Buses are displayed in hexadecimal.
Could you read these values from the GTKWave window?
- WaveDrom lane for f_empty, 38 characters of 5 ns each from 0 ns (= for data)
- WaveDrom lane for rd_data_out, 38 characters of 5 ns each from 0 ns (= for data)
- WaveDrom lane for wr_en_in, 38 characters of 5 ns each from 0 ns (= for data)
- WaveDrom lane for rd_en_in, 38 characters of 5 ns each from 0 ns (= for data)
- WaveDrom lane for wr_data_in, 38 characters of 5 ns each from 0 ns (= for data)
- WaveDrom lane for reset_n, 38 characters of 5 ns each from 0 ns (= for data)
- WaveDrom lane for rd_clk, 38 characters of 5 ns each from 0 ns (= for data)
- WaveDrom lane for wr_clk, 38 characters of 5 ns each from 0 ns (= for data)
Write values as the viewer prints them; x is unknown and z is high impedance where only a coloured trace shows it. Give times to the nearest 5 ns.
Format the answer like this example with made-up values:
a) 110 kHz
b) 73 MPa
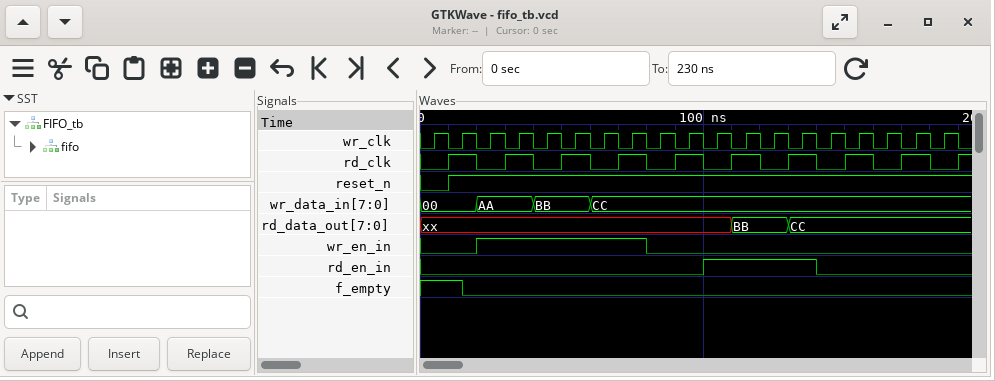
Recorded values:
a) {name: 'f_empty', wave: '1..0..................................'}
b) {name: 'rd_data_out', wave: 'x.....................=...=...........', data: 'BB CC'}
c) {name: 'wr_en_in', wave: '0...1...........0.....................'}
d) {name: 'rd_en_in', wave: '0...................1.......0.........'}
e) {name: 'wr_data_in', wave: '=...=...=...=.........................', data: '00 AA BB CC'}
f) {name: 'reset_n', wave: '0.1...................................'}
g) {name: 'rd_clk', wave: '0.1.0.1.0.1.0.1.0.1.0.1.0.1.0.1.0.1.0.'}
h) {name: 'wr_clk', wave: '01010101010101010101010101010101010101'}
